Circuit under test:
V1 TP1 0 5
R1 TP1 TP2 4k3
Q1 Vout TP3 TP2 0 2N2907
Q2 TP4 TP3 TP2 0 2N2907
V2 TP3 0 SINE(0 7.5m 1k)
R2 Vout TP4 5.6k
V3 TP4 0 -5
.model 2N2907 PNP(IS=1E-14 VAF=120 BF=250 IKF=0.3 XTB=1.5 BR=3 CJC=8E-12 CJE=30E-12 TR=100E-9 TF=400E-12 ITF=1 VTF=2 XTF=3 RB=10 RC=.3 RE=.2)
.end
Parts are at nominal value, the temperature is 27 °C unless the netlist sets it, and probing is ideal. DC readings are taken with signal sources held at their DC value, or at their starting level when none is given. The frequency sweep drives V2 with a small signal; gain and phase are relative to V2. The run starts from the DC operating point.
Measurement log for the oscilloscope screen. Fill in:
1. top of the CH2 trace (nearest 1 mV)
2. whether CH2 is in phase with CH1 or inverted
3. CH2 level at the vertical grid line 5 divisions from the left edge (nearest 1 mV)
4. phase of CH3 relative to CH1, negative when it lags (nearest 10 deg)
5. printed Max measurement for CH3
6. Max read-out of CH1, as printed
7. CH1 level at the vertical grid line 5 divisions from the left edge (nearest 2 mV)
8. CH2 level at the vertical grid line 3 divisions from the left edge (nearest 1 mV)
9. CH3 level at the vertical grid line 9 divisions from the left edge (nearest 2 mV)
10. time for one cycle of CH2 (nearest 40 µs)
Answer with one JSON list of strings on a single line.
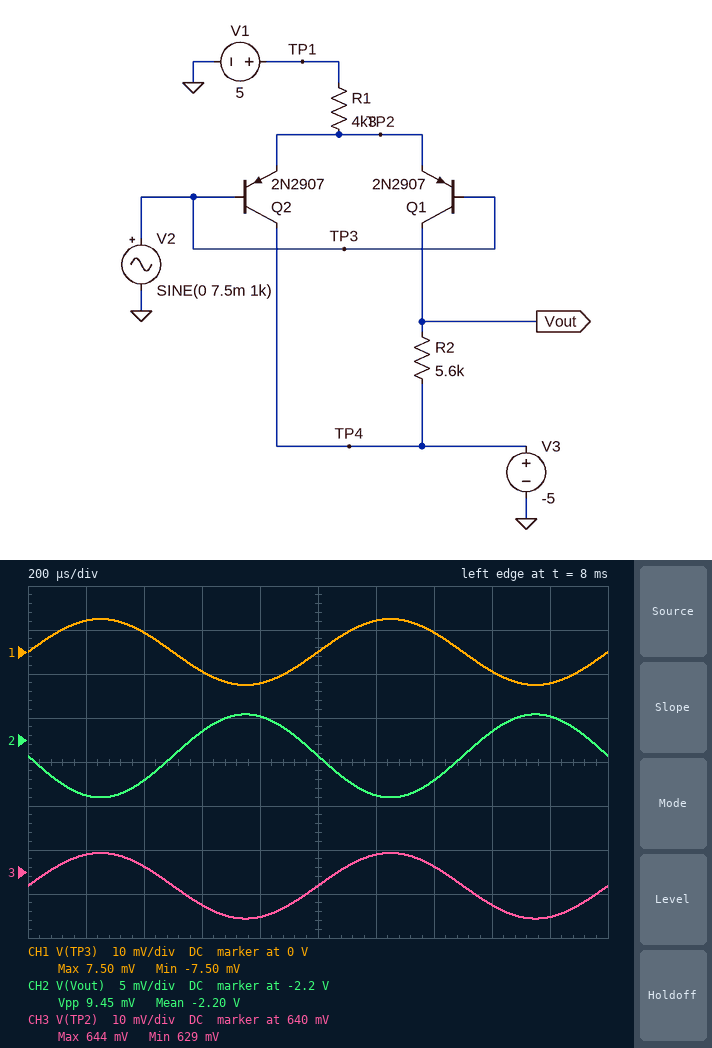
["-2.197 V", "inverted", "-2.202 V", "0 deg", "644 mV", "7.50 mV", "0 V", "-2.199 V", "630 mV", "1.00 ms"]
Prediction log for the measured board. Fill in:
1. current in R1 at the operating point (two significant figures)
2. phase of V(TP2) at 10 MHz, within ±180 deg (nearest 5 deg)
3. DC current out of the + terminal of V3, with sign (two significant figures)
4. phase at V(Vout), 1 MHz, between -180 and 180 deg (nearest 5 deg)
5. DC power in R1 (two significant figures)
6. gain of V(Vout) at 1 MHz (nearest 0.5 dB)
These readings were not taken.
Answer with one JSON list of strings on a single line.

["1.0 mA", "0 deg", "-1.0 mA", "150 deg", "4.4 mW", "-4.0 dB"]
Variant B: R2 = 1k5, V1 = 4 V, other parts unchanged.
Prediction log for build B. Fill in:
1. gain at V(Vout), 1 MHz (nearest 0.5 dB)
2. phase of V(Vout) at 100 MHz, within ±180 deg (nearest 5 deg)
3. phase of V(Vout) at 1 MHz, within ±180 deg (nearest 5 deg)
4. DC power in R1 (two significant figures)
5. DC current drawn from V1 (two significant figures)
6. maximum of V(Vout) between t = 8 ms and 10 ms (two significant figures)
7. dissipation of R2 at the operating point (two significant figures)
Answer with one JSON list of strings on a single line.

["-15.0 dB", "15 deg", "165 deg", "2.6 mW", "780 µA", "-4.4 V", "230 µW"]
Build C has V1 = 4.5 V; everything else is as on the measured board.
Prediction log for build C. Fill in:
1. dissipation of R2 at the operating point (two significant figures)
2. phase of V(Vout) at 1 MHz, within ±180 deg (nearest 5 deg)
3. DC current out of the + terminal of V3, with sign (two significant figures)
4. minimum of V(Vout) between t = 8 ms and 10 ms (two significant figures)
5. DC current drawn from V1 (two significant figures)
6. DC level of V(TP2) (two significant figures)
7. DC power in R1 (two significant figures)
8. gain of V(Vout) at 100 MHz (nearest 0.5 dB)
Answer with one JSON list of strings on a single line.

["1.1 mW", "155 deg", "-900 µA", "-2.5 V", "900 µA", "630 mV", "3.5 mW", "-0.5 dB"]
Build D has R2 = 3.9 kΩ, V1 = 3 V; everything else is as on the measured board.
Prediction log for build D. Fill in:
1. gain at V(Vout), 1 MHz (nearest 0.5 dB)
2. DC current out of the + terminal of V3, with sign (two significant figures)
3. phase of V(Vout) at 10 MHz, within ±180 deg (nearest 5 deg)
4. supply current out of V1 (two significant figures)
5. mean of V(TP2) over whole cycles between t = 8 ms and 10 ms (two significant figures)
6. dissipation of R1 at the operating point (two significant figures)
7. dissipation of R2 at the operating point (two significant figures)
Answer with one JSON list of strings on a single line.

["-7.0 dB", "-550 µA", "60 deg", "550 µA", "620 mV", "1.3 mW", "290 µW"]
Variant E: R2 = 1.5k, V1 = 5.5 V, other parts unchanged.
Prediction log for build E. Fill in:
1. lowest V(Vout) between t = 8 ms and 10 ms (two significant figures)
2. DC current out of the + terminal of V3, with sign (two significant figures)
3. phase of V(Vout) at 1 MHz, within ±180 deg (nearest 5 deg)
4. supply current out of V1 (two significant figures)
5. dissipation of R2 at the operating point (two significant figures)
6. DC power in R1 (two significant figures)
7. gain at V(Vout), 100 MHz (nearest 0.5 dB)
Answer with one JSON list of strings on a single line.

["-4.2 V", "-1.1 mA", "165 deg", "1.1 mA", "470 µW", "5.5 mW", "-1.0 dB"]
